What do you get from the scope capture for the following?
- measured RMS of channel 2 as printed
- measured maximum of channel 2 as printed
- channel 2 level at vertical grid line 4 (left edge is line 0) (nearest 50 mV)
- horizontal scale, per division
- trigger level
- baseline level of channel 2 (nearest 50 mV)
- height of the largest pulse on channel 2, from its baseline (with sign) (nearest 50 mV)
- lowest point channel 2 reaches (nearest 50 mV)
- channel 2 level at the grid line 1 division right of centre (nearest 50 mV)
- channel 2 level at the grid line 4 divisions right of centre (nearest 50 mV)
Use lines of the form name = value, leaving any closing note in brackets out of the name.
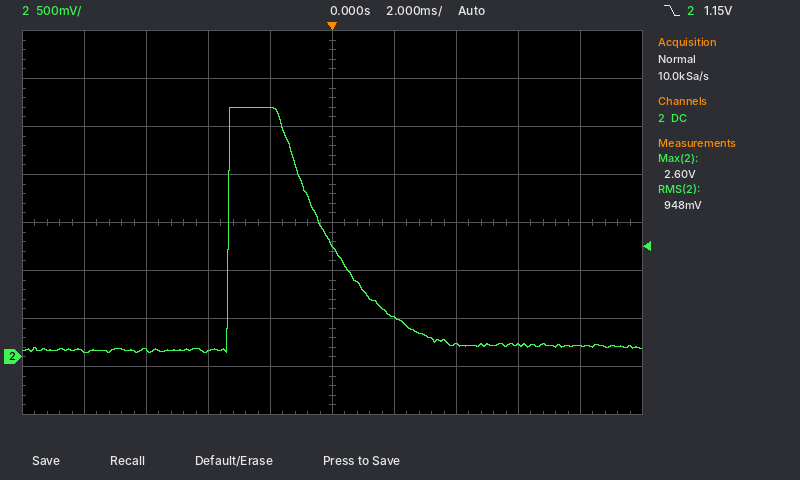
measured RMS of channel 2 as printed = 948 mV
measured maximum of channel 2 as printed = 2.60 V
channel 2 level at vertical grid line 4 (left edge is line 0) = 2.60 V
horizontal scale, per division = 2 ms
trigger level = 1.15 V
baseline level of channel 2 = 100 mV
height of the largest pulse on channel 2, from its baseline (with sign) = +2.50 V
lowest point channel 2 reaches = 50 mV
channel 2 level at the grid line 1 division right of centre = 400 mV
channel 2 level at the grid line 4 divisions right of centre = 100 mV
